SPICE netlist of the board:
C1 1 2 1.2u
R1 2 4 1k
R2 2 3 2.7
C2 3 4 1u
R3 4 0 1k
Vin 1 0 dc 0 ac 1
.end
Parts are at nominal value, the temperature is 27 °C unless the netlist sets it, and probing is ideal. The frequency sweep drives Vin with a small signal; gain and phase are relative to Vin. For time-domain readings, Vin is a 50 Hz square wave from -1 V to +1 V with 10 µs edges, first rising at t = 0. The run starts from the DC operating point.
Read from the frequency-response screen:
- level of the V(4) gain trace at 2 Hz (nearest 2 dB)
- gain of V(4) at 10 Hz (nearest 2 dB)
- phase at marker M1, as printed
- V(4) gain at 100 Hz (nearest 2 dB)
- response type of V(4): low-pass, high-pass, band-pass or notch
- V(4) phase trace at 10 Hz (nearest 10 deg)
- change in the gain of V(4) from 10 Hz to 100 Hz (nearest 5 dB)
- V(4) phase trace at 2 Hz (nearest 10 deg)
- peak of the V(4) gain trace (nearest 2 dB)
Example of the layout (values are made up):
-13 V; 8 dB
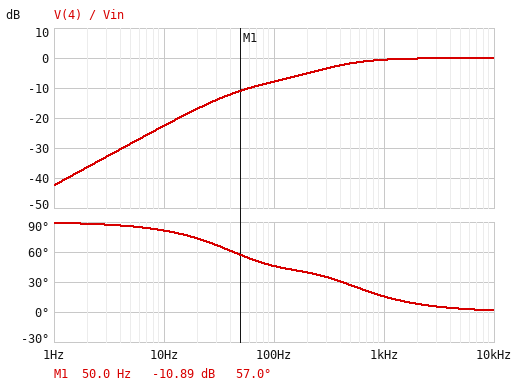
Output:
-36 dB; -22 dB; 57.0 deg; -8 dB; high-pass; 80 deg; 15 dB; 90 deg; 0 dB
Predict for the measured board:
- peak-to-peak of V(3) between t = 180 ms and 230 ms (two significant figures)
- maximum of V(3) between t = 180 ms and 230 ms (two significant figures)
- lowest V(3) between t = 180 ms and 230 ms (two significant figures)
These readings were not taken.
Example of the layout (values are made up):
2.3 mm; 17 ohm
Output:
3.9 V; 1.9 V; -1.9 V
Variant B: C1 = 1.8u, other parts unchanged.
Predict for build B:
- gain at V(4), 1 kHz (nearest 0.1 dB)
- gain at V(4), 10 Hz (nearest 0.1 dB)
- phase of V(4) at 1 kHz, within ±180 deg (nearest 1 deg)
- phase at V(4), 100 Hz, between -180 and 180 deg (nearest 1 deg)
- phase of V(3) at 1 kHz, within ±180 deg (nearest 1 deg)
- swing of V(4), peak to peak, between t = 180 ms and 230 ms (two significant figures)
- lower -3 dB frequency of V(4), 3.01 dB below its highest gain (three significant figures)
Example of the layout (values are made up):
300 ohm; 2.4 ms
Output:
-0.5 dB; -19.2 dB; 13 deg; 38 deg; 5 deg; 3.8 V; 296 Hz
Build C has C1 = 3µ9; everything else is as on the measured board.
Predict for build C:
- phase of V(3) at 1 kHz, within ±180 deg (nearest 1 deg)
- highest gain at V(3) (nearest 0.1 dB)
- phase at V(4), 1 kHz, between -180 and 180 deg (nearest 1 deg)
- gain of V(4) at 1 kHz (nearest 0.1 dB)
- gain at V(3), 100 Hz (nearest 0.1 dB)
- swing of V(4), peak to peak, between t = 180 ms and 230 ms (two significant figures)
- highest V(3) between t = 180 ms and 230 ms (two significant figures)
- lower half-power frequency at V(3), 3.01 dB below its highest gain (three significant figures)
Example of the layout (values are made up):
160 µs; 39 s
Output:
2 deg; 0 dB; 11 deg; -0.4 dB; -0.7 dB; 3.6 V; 1.6 V; 21.9 Hz
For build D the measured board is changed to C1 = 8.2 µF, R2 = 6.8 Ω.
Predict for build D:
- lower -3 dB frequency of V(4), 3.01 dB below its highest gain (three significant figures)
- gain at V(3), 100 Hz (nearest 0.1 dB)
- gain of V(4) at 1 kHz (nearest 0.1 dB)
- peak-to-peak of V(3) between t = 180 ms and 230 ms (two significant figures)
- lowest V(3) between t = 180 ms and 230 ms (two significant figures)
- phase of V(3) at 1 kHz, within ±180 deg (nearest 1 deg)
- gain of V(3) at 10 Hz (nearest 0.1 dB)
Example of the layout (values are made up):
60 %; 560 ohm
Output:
235 Hz; -0.3 dB; -0.4 dB; 2.6 V; -1.3 V; 1 deg; -3.0 dB
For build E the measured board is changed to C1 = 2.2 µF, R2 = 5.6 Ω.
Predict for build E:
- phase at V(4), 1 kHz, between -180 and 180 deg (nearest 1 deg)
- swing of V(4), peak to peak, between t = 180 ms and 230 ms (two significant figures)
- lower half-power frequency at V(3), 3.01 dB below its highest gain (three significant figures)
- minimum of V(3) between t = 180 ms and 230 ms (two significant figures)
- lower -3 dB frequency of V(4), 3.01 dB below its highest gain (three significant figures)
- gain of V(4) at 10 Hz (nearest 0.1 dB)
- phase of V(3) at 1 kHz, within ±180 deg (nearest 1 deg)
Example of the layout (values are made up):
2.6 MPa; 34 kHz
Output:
12 deg; 3.8 V; 41.5 Hz; -1.8 V; 280 Hz; -17.6 dB; 4 deg
